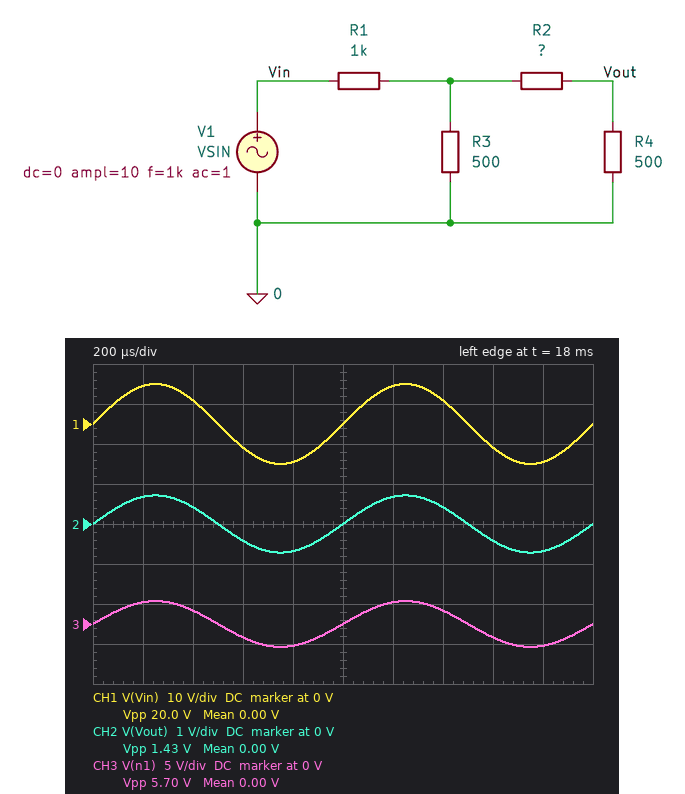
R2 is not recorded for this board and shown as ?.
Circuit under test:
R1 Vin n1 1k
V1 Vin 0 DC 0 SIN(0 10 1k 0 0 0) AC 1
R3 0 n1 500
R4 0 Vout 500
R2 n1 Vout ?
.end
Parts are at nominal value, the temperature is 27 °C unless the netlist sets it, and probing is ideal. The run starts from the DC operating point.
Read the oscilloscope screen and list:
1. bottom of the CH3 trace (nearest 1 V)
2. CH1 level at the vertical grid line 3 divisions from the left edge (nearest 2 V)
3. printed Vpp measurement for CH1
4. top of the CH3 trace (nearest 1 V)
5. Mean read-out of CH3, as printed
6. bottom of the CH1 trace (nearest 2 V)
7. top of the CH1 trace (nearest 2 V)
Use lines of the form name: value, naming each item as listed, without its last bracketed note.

bottom of the CH3 trace: -3 V
CH1 level at the vertical grid line 3 divisions from the left edge: -6 V
printed Vpp measurement for CH1: 20.0 V
top of the CH3 trace: 3 V
Mean read-out of CH3, as printed: 0.00 V
bottom of the CH1 trace: -10 V
top of the CH1 trace: 10 V
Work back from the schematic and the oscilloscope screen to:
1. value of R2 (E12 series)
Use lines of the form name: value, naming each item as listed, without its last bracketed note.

value of R2: 1.5 kΩ
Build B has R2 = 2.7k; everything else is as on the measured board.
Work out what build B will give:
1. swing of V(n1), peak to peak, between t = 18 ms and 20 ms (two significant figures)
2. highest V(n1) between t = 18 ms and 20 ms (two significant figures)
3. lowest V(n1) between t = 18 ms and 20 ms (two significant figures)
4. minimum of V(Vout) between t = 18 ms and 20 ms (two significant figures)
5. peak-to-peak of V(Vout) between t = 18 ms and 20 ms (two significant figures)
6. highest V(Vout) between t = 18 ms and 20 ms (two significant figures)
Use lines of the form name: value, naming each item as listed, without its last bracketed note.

swing of V(n1), peak to peak, between t = 18 ms and 20 ms: 6.0 V
highest V(n1) between t = 18 ms and 20 ms: 3.0 V
lowest V(n1) between t = 18 ms and 20 ms: -3.0 V
minimum of V(Vout) between t = 18 ms and 20 ms: -470 mV
peak-to-peak of V(Vout) between t = 18 ms and 20 ms: 940 mV
highest V(Vout) between t = 18 ms and 20 ms: 470 mV
